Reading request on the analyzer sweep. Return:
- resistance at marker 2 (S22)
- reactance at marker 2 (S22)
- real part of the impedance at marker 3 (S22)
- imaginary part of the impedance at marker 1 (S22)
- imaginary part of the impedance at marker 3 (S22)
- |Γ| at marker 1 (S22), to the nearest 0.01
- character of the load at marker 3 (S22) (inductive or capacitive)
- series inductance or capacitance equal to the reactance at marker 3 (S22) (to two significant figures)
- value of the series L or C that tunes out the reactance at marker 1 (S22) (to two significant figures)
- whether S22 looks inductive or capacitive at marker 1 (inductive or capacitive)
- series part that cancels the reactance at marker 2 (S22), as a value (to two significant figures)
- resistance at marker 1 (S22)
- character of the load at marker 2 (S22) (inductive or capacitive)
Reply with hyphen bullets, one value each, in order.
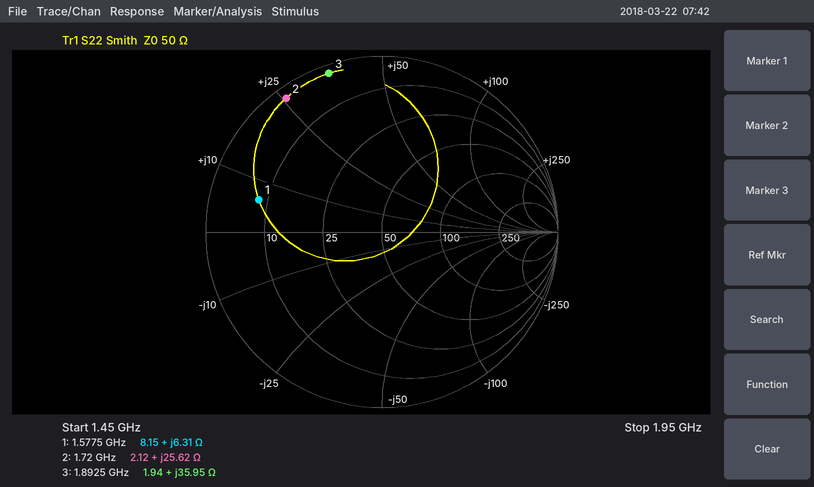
- 2.12 Ω
- +25.62 Ω
- 1.94 Ω
- +6.31 Ω
- +35.95 Ω
- 0.72
- inductive
- 3.0 nH
- 16 pF
- inductive
- 3.6 pF
- 8.15 Ω
- inductive
